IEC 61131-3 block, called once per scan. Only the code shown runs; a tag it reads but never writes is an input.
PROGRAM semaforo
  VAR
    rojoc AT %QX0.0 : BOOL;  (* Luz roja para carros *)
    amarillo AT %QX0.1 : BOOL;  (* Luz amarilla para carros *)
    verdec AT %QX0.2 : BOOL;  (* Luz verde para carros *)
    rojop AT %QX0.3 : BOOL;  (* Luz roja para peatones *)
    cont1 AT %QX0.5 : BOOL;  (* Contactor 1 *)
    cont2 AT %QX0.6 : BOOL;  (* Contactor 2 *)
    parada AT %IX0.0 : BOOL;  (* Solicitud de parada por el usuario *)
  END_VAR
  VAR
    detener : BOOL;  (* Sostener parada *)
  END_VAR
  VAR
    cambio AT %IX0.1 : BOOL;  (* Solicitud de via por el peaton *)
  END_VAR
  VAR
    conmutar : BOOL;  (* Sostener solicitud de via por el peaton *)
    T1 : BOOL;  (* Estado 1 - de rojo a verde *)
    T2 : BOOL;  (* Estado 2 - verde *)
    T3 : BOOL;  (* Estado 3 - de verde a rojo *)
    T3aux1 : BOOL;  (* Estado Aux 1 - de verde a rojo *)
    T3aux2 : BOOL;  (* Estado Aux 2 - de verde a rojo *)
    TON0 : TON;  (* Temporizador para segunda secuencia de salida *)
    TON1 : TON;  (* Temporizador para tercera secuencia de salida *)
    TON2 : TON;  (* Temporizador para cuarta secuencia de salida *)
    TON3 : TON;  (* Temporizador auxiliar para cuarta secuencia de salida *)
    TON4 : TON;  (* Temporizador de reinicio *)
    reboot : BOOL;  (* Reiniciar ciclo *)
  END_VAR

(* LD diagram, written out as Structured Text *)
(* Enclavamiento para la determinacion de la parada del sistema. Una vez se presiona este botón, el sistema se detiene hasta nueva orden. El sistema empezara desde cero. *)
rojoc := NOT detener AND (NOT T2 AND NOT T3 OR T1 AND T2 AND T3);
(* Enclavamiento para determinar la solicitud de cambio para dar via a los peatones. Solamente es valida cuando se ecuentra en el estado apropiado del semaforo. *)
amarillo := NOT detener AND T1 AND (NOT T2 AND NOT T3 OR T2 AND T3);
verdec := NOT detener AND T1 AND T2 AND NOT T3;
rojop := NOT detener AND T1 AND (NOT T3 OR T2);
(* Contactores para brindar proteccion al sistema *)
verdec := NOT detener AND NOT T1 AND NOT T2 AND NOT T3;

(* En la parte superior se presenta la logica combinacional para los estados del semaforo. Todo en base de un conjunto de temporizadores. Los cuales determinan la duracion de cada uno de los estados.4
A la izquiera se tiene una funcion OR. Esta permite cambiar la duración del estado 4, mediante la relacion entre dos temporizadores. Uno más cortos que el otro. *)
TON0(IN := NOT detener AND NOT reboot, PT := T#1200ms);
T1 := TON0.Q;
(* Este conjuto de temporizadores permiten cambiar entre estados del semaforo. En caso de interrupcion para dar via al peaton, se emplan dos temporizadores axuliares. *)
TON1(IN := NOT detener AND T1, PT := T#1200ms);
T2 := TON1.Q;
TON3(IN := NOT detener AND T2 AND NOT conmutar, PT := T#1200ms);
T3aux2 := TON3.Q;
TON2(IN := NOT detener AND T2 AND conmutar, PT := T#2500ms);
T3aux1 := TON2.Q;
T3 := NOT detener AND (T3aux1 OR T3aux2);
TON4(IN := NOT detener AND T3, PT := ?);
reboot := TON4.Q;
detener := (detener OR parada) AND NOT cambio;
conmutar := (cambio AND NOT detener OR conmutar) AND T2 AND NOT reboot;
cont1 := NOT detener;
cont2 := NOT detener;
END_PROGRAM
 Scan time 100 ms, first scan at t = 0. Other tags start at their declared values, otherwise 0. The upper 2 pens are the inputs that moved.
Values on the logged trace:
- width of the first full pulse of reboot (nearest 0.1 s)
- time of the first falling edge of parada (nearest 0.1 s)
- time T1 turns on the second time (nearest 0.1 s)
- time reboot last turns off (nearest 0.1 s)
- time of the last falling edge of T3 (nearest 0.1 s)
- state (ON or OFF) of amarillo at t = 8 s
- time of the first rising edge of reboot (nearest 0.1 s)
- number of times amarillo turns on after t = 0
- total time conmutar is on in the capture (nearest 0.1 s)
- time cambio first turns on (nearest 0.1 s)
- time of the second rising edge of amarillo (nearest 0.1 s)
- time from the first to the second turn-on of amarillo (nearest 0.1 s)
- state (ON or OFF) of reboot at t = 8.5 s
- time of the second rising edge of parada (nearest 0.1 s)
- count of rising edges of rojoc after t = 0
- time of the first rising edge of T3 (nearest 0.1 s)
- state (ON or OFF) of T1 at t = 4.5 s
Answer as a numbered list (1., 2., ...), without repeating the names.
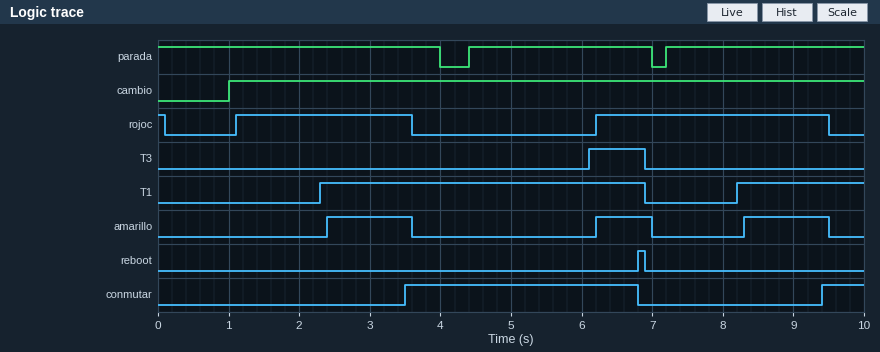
1. 0.1 s
2. 4.0 s
3. 8.2 s
4. 6.9 s
5. 6.9 s
6. OFF
7. 6.8 s
8. 3
9. 3.9 s
10. 1.0 s
11. 6.2 s
12. 3.8 s
13. OFF
14. 7.2 s
15. 2
16. 6.1 s
17. ON
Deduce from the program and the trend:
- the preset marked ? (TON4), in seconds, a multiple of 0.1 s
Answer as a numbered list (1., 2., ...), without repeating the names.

1. 0.7 s
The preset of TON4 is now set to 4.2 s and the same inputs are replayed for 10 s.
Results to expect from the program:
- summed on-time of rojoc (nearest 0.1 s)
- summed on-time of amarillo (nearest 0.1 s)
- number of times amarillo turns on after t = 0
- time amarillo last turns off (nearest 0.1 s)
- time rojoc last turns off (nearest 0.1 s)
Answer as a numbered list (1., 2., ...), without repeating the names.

1. 6.4 s
2. 5.0 s
3. 2
4. 3.6 s
5. 3.6 s
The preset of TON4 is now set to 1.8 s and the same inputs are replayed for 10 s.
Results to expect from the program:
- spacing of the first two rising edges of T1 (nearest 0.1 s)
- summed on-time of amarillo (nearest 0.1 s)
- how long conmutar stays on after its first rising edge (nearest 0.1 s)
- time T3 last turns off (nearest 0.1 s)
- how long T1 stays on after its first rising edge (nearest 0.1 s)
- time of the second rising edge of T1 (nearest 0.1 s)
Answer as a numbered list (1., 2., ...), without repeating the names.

1. 7.0 s
2. 3.7 s
3. 4.4 s
4. 8.0 s
5. 5.7 s
6. 9.3 s
